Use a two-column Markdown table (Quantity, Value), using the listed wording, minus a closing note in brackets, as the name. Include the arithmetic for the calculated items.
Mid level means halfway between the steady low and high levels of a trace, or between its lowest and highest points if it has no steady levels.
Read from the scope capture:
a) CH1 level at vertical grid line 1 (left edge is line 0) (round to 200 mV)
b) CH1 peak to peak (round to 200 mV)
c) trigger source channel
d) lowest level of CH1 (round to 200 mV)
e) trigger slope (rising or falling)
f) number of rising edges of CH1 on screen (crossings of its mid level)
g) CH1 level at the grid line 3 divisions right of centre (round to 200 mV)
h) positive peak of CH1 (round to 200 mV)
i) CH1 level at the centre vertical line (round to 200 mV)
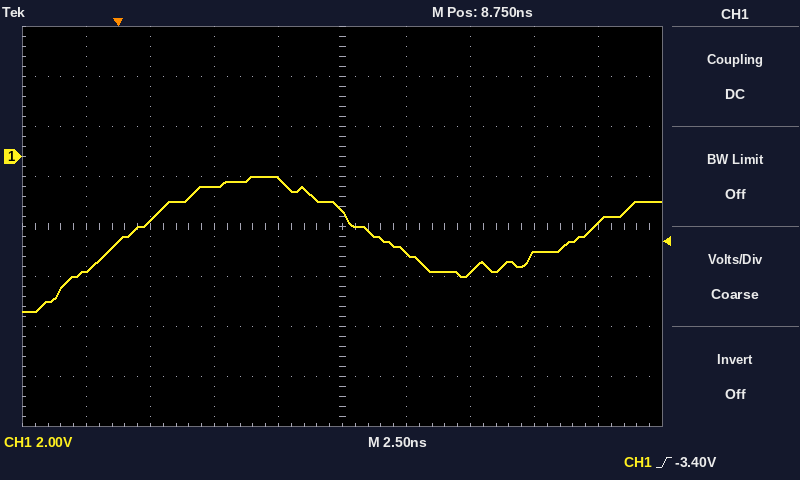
| Quantity | Value |
|---|---|
| CH1 level at vertical grid line 1 (left edge is line 0) | -4.6 V |
| CH1 peak to peak | -800 mV − (-6.2 V) = 5.4 V |
| trigger source channel | CH1 |
| lowest level of CH1 | -6.2 V |
| trigger slope | rising |
| number of rising edges of CH1 on screen | 2 |
| CH1 level at the grid line 3 divisions right of centre | -3.8 V |
| positive peak of CH1 | -800 mV |
| CH1 level at the centre vertical line | -2.2 V |
